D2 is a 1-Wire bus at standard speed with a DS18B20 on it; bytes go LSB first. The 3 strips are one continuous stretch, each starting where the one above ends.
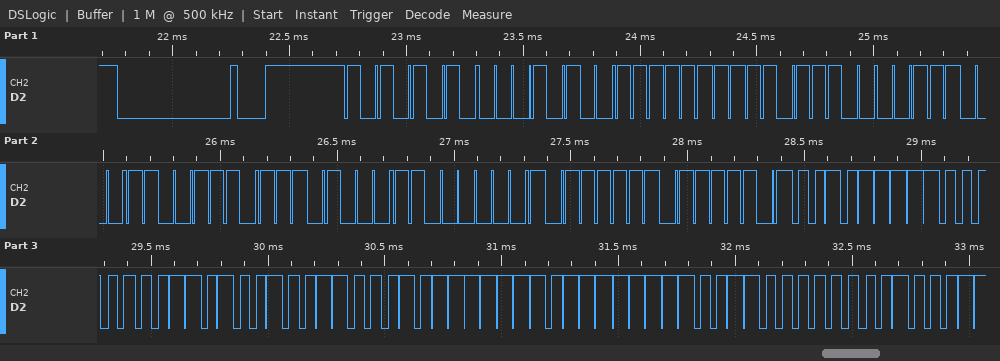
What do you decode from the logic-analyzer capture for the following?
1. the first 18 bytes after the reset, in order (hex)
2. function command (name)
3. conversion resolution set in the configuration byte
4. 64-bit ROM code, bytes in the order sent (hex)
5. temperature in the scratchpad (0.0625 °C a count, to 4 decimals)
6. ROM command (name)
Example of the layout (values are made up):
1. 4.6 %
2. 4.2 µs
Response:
1. 55 28 FF 3B 1C 73 17 03 FD BE F4 01 4B 46 7F FF 0C 10
2. Read Scratchpad
3. 12 bits
4. 28 FF 3B 1C 73 17 03 FD
5. 31.2500 °C
6. Match ROM
